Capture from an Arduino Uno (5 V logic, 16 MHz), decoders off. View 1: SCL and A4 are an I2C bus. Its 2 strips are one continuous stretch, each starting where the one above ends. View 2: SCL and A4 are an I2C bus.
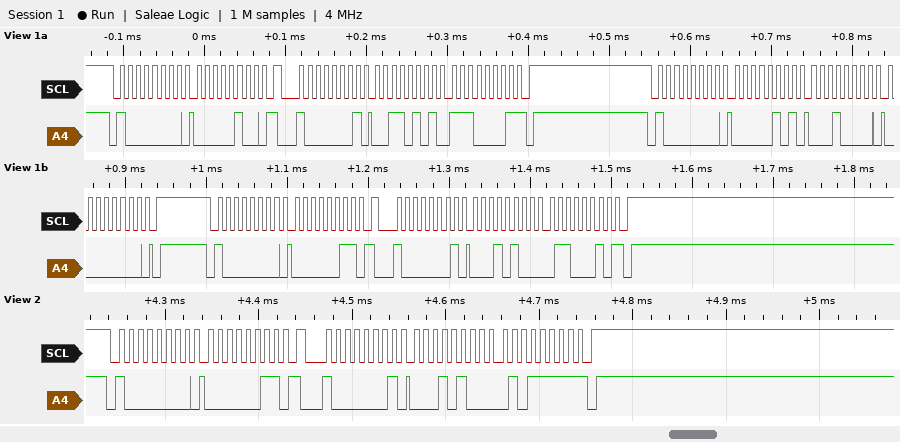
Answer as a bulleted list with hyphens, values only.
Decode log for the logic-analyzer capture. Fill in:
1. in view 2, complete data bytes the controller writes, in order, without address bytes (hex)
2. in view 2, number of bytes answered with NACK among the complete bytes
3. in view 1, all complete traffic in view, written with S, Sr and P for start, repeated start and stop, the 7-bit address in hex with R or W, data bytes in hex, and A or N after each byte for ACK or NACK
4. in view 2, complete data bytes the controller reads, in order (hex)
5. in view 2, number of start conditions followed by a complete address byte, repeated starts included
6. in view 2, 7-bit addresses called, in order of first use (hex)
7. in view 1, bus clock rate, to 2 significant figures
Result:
- 03
- 1
- S 40W A 04 A Sr 40R A 35 A E1 N P S 40W A 05 A 10 A 00 A P S 40W A 03 A Sr 40R A 14 A 62 N P
- 14 5F
- 2
- 0x40
- 100 kHz
